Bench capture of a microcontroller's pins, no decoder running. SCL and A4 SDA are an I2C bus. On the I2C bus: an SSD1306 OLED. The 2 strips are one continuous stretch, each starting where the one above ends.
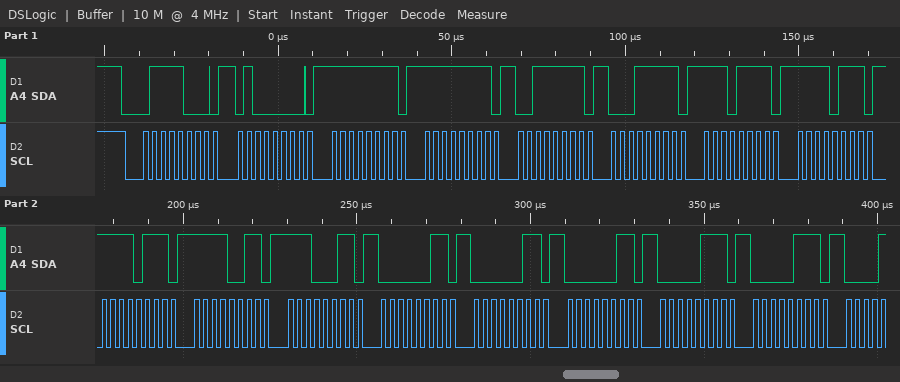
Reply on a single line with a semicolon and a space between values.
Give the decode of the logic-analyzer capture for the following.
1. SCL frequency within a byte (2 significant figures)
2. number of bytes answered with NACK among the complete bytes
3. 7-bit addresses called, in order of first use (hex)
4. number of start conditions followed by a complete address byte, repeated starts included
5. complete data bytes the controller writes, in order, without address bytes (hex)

400 kHz; 0; 0x3C; 1; 40 FF FF 3F 1F EF F7 F7 F3 E3 03 03 03 07 07
